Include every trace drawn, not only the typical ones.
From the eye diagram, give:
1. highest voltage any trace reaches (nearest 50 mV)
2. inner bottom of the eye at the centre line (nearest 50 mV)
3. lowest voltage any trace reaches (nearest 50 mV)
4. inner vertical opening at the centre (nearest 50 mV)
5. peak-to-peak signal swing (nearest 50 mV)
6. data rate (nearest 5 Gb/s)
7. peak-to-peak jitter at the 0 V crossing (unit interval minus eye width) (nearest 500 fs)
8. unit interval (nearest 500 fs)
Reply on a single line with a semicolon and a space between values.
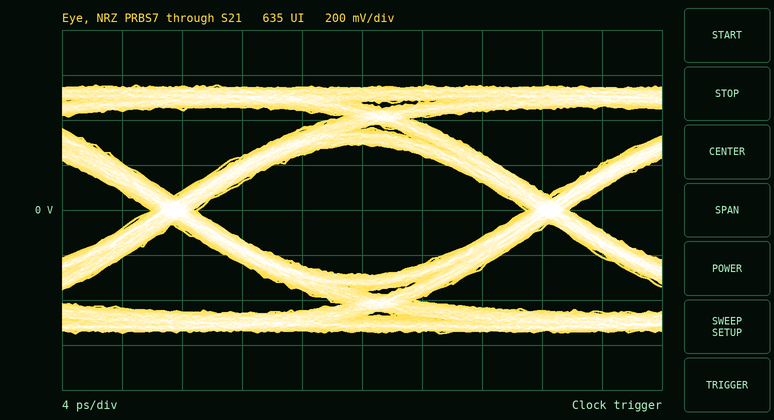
550 mV; -300 mV; -550 mV; 600 mV; 1.10 V; 40 Gb/s; 3.0 ps; 25.0 ps
